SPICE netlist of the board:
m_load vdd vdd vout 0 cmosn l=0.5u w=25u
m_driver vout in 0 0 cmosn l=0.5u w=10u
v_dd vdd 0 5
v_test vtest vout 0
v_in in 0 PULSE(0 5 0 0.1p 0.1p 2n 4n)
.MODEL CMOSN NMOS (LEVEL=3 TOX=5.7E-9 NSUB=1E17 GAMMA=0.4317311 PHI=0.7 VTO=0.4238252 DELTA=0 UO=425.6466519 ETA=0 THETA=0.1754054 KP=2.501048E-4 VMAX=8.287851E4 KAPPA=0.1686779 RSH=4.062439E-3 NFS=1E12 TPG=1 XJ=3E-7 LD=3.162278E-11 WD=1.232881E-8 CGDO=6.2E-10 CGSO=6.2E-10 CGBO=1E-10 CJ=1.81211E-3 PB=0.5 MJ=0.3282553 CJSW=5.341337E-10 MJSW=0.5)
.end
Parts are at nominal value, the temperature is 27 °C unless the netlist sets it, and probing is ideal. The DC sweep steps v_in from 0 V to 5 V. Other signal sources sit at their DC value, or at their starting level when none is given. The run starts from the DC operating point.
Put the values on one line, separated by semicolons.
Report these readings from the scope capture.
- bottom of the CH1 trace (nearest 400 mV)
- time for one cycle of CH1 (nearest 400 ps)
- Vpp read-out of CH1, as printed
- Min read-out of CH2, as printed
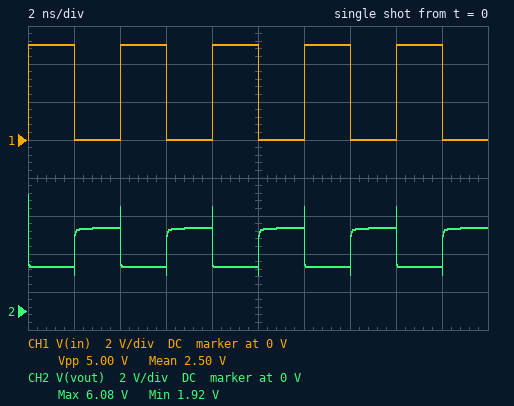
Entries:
0 V; 4.0 ns; 5.00 V; 1.92 V
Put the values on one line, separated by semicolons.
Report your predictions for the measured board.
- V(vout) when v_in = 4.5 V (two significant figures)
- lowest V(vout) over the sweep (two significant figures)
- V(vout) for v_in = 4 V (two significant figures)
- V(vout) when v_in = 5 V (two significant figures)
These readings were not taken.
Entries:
2.5 V; 2.3 V; 2.7 V; 2.3 V
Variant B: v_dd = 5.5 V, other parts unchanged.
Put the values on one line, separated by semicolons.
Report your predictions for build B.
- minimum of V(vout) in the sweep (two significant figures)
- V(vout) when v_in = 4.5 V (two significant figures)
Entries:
2.8 V; 3.0 V
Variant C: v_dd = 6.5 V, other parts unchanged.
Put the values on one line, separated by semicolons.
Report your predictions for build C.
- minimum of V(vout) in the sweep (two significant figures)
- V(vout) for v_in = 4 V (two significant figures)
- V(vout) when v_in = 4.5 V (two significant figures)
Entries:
3.7 V; 4.1 V; 3.9 V
